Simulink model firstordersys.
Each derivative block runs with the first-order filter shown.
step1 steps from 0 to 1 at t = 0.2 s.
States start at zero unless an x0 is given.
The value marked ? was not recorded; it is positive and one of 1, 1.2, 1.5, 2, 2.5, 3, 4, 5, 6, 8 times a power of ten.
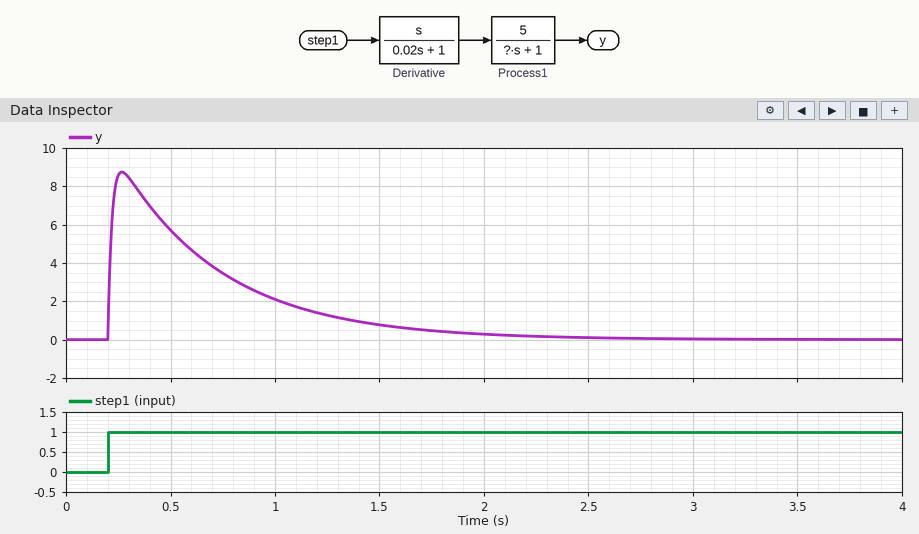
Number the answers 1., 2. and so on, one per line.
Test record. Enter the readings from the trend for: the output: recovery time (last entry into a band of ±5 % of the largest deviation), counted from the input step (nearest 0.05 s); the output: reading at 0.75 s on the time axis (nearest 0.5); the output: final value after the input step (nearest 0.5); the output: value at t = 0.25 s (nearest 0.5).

1. 1.60 s
2. 3.5
3. 0.0
4. 8.5
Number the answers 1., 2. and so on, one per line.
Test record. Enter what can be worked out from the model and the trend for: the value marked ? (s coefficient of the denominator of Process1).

1. 0.5
